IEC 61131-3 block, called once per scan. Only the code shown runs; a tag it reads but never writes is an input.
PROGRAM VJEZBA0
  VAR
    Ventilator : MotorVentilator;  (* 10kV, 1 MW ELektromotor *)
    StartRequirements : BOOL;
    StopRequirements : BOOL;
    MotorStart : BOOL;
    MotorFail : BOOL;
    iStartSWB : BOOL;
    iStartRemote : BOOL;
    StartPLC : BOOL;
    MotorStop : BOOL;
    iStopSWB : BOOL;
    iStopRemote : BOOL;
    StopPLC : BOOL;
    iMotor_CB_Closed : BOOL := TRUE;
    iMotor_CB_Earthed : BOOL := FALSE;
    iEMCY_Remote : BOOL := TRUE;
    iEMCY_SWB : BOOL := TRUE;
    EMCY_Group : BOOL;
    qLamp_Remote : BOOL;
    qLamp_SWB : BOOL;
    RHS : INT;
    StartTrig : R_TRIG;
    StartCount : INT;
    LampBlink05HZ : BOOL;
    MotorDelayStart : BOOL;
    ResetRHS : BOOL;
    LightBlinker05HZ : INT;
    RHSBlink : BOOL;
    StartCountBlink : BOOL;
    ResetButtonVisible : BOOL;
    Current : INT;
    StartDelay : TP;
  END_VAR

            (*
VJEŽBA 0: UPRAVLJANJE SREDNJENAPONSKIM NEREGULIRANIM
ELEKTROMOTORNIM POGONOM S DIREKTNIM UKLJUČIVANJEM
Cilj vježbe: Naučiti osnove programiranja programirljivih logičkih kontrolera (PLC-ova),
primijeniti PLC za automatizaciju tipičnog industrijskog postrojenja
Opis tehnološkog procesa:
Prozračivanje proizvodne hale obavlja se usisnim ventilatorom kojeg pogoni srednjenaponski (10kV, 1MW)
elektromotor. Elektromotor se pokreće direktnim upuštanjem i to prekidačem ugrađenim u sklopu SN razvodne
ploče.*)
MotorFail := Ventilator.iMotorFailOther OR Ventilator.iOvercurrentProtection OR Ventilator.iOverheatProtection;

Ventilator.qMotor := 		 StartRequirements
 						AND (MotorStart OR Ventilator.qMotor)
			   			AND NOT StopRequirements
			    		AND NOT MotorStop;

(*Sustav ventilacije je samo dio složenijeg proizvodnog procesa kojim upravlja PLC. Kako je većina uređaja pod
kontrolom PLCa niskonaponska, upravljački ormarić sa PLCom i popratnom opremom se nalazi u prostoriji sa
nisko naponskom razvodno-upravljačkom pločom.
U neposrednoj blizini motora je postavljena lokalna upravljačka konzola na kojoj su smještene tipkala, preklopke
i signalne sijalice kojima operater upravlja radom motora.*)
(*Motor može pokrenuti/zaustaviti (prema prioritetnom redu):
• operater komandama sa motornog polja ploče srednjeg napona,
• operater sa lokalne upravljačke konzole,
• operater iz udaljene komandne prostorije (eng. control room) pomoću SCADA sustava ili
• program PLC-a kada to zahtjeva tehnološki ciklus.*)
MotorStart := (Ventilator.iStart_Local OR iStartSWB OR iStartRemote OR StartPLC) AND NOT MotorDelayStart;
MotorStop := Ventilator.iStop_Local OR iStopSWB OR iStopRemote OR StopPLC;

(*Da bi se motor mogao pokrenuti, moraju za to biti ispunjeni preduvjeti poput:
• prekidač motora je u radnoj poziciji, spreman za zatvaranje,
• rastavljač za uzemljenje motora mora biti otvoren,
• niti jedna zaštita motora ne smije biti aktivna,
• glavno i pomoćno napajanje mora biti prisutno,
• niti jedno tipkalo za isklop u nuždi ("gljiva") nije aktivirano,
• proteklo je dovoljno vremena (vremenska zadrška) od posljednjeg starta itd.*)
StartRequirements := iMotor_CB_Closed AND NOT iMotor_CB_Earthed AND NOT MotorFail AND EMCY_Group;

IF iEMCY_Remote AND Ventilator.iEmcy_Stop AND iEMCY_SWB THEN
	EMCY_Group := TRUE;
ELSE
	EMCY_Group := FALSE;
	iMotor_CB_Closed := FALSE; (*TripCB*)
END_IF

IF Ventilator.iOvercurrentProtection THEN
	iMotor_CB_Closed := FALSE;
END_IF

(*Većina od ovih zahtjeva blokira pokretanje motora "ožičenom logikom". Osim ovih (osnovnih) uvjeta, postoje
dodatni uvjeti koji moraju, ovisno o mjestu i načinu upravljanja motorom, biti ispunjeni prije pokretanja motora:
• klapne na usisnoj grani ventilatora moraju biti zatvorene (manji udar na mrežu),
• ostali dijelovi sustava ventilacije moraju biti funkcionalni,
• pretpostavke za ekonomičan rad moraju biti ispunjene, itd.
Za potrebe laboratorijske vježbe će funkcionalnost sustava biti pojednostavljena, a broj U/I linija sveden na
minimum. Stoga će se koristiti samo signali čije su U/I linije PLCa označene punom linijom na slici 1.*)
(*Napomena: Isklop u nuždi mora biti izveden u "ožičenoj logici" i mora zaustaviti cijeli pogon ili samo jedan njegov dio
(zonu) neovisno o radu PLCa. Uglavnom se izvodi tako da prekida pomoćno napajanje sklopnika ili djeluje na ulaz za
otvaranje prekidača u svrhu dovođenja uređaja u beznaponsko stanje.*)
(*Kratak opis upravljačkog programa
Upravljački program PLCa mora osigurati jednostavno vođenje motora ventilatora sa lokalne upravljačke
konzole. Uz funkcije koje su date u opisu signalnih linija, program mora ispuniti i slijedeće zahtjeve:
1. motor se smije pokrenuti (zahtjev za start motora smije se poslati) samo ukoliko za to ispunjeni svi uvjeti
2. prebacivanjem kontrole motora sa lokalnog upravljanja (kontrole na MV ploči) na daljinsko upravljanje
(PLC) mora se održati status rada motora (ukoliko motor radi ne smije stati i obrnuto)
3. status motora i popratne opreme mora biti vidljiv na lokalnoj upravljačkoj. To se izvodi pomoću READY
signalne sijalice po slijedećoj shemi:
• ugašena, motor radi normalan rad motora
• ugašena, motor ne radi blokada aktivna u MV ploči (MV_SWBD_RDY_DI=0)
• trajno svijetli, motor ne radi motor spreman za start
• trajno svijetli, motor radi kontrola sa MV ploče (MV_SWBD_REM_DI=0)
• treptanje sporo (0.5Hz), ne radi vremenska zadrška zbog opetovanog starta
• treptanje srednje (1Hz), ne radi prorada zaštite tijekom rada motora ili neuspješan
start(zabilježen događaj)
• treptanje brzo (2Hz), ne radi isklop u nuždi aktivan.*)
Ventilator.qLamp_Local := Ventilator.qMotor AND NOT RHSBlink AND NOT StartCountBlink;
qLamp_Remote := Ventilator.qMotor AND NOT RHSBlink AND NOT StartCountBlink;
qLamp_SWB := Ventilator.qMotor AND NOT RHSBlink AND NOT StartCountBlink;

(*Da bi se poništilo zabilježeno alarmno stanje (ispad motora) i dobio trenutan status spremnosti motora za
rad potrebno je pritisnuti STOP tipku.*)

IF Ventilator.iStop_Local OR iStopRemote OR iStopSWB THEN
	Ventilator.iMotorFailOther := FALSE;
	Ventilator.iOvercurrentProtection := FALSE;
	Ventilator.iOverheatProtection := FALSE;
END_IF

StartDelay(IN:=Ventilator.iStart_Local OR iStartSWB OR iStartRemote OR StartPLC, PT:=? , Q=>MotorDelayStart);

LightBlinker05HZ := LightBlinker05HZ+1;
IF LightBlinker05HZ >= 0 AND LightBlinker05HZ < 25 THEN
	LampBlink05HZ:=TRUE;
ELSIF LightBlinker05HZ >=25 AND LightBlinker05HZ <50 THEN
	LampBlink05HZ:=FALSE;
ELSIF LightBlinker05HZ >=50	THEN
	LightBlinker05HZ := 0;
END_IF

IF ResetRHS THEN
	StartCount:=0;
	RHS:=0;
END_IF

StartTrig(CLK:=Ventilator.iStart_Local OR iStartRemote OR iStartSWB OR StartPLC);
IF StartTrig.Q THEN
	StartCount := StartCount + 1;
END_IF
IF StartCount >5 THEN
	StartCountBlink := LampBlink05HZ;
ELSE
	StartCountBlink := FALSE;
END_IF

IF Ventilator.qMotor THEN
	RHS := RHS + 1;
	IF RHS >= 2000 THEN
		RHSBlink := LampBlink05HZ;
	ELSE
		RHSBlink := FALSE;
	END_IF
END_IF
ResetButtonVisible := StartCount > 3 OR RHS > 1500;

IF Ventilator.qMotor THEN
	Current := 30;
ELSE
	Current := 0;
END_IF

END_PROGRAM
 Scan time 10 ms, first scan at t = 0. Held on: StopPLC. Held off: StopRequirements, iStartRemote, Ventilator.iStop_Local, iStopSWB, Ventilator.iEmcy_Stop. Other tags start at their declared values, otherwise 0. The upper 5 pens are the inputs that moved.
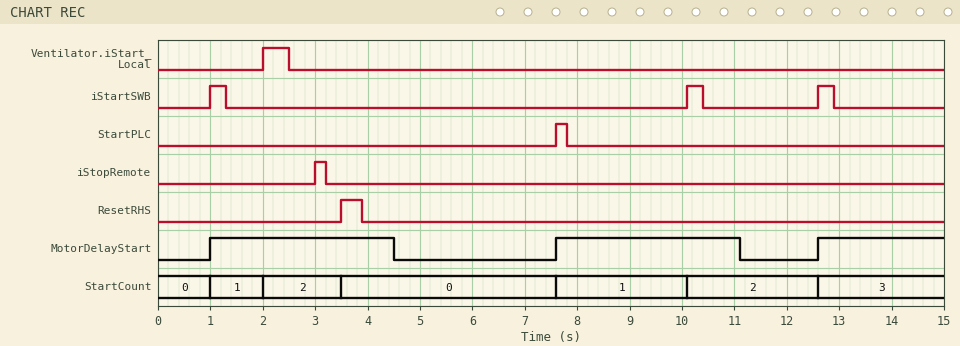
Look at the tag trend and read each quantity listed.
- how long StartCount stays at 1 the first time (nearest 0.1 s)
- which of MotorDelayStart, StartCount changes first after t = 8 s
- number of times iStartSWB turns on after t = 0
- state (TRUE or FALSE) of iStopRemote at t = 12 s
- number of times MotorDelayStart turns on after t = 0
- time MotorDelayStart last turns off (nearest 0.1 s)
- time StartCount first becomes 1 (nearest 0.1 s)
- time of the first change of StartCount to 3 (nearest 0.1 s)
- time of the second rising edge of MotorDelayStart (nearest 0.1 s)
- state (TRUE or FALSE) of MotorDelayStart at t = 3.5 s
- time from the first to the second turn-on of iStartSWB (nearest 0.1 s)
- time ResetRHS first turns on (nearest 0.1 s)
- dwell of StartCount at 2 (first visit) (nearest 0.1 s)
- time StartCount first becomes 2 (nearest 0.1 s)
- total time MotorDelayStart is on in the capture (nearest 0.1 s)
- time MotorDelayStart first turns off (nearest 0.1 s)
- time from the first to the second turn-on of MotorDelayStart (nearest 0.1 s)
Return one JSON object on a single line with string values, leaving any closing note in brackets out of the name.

{"how long StartCount stays at 1 the first time": "1.0 s", "which of MotorDelayStart, StartCount changes first after t = 8 s": "StartCount", "number of times iStartSWB turns on after t = 0": "3", "state (TRUE or FALSE) of iStopRemote at t = 12 s": "FALSE", "number of times MotorDelayStart turns on after t = 0": "3", "time MotorDelayStart last turns off": "11.1 s", "time StartCount first becomes 1": "1.0 s", "time of the first change of StartCount to 3": "12.6 s", "time of the second rising edge of MotorDelayStart": "7.6 s", "state (TRUE or FALSE) of MotorDelayStart at t = 3.5 s": "TRUE", "time from the first to the second turn-on of iStartSWB": "9.1 s", "time ResetRHS first turns on": "3.5 s", "dwell of StartCount at 2 (first visit)": "1.5 s", "time StartCount first becomes 2": "2.0 s", "total time MotorDelayStart is on in the capture": "9.4 s", "time MotorDelayStart first turns off": "4.5 s", "time from the first to the second turn-on of MotorDelayStart": "6.6 s"}
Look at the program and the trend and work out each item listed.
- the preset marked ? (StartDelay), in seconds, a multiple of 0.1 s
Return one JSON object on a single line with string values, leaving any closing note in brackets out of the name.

{"the preset marked ? (StartDelay), in seconds, a multiple of 0.1 s": "3.5 s"}
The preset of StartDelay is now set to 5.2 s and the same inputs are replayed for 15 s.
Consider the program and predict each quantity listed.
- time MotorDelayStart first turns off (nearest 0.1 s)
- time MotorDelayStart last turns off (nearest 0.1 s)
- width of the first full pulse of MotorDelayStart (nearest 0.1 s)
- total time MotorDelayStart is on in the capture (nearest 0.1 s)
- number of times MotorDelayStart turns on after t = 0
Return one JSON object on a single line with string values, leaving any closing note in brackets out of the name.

{"time MotorDelayStart first turns off": "6.2 s", "time MotorDelayStart last turns off": "12.8 s", "width of the first full pulse of MotorDelayStart": "5.2 s", "total time MotorDelayStart is on in the capture": "10.4 s", "number of times MotorDelayStart turns on after t = 0": "2"}
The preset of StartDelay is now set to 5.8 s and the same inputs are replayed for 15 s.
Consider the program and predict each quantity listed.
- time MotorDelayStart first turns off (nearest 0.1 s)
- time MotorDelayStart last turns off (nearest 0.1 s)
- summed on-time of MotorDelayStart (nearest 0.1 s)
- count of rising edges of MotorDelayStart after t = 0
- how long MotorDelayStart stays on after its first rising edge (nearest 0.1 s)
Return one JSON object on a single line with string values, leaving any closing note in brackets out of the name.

{"time MotorDelayStart first turns off": "6.8 s", "time MotorDelayStart last turns off": "13.4 s", "summed on-time of MotorDelayStart": "11.6 s", "count of rising edges of MotorDelayStart after t = 0": "2", "how long MotorDelayStart stays on after its first rising edge": "5.8 s"}
